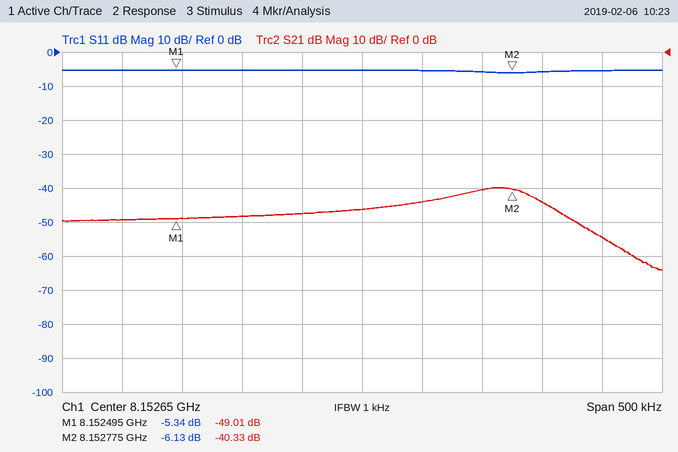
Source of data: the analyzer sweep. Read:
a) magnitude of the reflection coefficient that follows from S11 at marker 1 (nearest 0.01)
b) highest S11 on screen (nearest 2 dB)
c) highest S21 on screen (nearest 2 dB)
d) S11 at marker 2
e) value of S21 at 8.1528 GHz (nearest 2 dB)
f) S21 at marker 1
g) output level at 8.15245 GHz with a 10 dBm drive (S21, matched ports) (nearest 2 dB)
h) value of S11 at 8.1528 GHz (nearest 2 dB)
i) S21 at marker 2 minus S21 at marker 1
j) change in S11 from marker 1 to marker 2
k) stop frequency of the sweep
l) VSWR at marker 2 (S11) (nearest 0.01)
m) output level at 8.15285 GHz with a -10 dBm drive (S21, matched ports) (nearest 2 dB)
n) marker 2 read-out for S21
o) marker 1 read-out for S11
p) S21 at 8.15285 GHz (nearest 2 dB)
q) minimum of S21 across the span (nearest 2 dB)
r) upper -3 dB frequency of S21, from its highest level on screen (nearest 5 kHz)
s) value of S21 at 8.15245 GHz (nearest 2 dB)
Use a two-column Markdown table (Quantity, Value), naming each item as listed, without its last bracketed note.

| Quantity | Value |
|---|---|
| magnitude of the reflection coefficient that follows from S11 at marker 1 | 0.54 |
| highest S11 on screen | -6 dB |
| highest S21 on screen | -40 dB |
| S11 at marker 2 | -6.13 dB |
| value of S21 at 8.1528 GHz | -44 dB |
| S21 at marker 1 | -49.01 dB |
| output level at 8.15245 GHz with a 10 dBm drive (S21, matched ports) | -40 dBm |
| value of S11 at 8.1528 GHz | -6 dB |
| S21 at marker 2 minus S21 at marker 1 | 8.68 dB |
| change in S11 from marker 1 to marker 2 | -0.79 dB |
| stop frequency of the sweep | 8.1529 GHz |
| VSWR at marker 2 (S11) | 2.95 |
| output level at 8.15285 GHz with a -10 dBm drive (S21, matched ports) | -64 dBm |
| marker 2 read-out for S21 | -40.33 dB |
| marker 1 read-out for S11 | -5.34 dB |
| S21 at 8.15285 GHz | -54 dB |
| minimum of S21 across the span | -64 dB |
| upper -3 dB frequency of S21, from its highest level on screen | 8.152795 GHz |
| value of S21 at 8.15245 GHz | -50 dB |
